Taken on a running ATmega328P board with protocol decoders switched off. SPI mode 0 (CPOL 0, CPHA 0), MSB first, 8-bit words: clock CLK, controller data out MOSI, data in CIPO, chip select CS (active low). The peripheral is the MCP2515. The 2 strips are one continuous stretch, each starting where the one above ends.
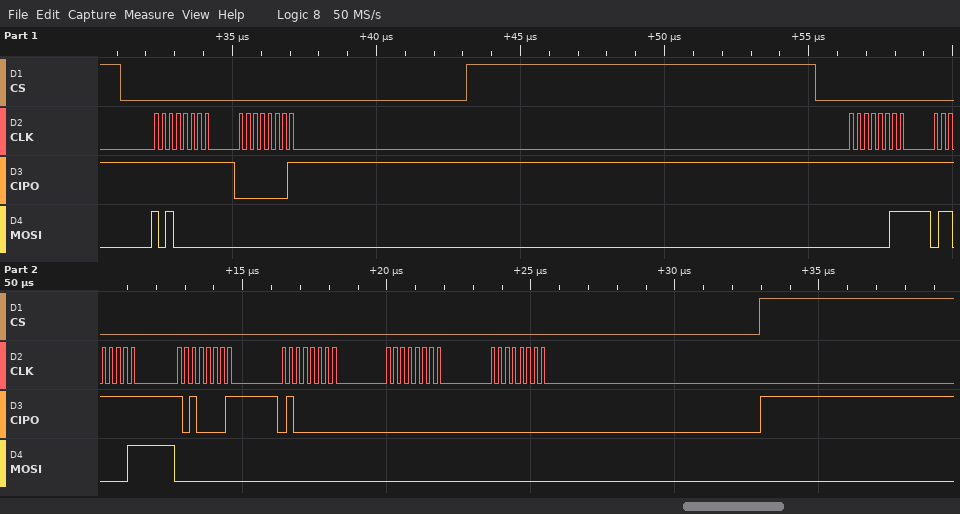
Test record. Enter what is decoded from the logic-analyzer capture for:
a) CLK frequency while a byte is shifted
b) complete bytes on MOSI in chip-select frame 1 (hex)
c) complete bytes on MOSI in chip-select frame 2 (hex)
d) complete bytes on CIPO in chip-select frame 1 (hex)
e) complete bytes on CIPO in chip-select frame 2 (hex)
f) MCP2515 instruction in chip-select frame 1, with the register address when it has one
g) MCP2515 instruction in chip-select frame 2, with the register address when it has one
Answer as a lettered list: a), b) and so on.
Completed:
a) 4 MHz
b) 0xA0 0x00
c) 0x03 0x61 0x00 0x00 0x00 0x00
d) 0xFF 0x01
e) 0xFF 0xFF 0xA1 0x40 0x00 0x00
f) READ STATUS
g) READ 0x61
